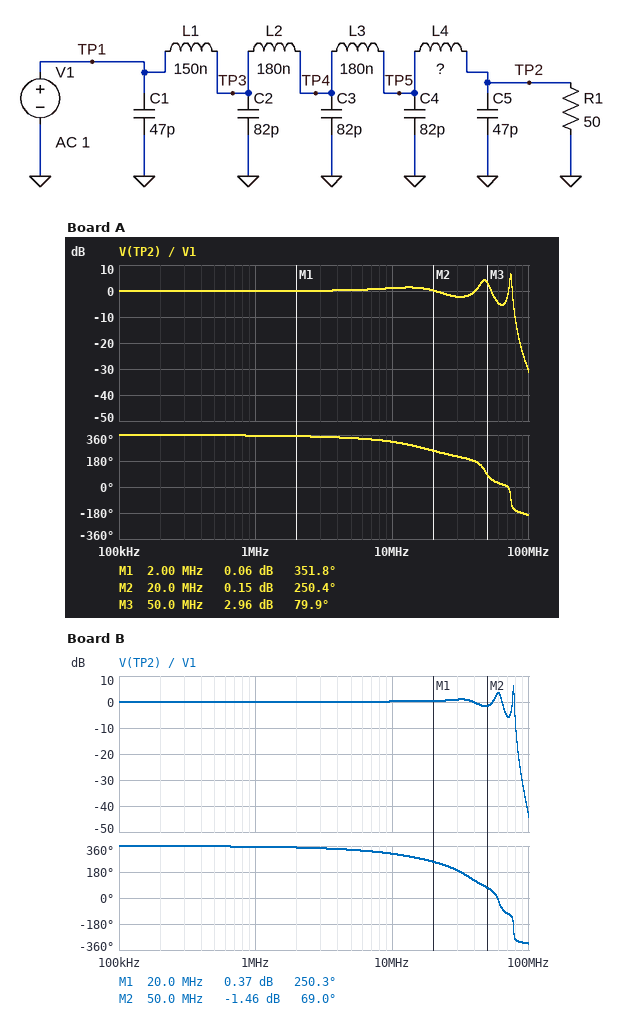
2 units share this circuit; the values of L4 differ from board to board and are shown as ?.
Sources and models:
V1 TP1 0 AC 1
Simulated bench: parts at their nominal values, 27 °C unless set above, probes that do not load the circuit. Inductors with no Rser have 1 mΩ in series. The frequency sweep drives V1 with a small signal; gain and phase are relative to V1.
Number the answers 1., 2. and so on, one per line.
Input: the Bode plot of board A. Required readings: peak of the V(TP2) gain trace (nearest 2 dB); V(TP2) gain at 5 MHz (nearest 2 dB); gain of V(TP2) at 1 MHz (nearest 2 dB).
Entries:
1. 6 dB
2. 0 dB
3. 0 dB
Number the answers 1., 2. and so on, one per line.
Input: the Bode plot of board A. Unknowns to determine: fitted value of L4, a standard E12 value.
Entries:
1. 56 nH
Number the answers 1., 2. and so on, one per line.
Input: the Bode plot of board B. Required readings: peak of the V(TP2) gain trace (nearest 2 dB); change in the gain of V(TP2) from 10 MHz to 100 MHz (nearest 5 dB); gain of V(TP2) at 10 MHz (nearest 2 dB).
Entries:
1. 6 dB
2. -45 dB
3. 0 dB
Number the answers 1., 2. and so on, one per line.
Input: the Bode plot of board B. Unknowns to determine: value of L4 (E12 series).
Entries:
1. 220 nH
